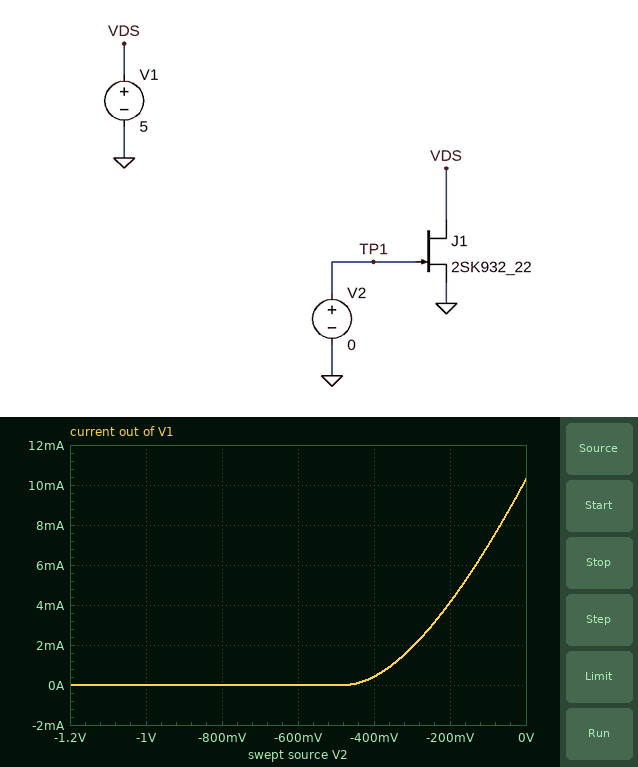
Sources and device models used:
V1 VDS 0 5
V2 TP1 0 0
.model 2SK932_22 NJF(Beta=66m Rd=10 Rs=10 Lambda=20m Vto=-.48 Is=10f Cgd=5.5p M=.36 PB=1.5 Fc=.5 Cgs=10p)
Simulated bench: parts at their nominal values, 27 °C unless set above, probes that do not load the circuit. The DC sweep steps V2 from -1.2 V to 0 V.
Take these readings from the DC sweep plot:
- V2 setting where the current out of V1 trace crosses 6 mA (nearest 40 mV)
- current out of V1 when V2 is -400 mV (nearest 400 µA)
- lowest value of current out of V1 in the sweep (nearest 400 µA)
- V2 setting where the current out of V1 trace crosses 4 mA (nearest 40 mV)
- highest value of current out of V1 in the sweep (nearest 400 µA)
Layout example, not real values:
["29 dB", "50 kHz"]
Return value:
["-120 mV", "400 µA", "0 A", "-200 mV", "10.4 mA"]
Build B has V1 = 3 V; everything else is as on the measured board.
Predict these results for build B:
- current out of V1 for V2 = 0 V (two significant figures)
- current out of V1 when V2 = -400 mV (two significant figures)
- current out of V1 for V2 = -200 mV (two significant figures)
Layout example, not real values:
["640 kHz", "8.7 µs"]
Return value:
["10 mA", "400 µA", "4.0 mA"]
